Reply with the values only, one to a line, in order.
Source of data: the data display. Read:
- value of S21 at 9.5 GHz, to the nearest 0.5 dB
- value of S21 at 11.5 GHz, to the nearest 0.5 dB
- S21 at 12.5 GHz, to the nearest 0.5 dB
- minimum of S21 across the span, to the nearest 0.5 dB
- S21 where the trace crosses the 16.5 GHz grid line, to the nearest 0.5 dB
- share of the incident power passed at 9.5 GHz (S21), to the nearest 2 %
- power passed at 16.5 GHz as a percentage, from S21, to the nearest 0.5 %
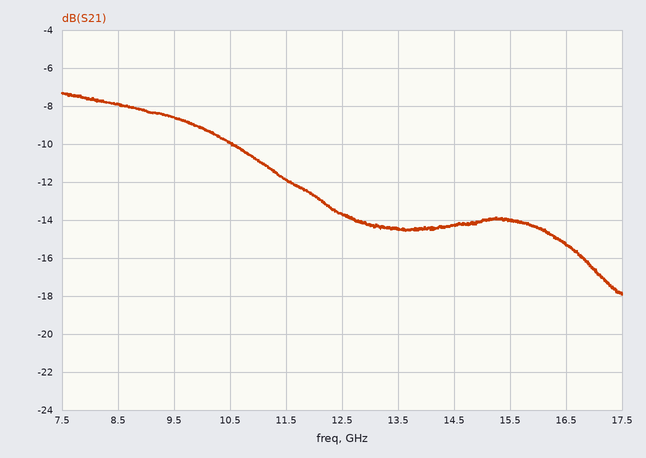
-8.5 dB
-12.0 dB
-13.5 dB
-18.0 dB
-15.5 dB
14 %
3.0 %
